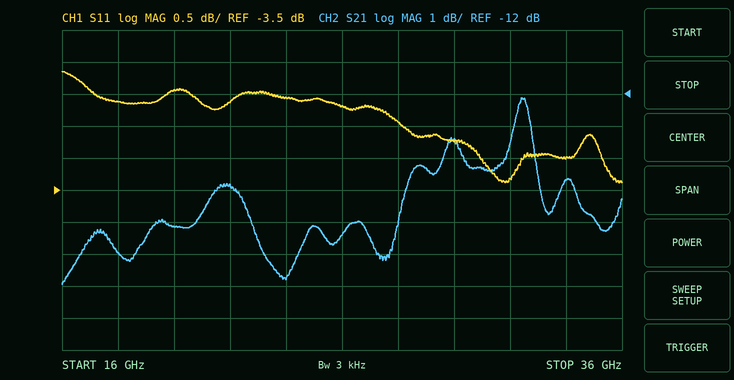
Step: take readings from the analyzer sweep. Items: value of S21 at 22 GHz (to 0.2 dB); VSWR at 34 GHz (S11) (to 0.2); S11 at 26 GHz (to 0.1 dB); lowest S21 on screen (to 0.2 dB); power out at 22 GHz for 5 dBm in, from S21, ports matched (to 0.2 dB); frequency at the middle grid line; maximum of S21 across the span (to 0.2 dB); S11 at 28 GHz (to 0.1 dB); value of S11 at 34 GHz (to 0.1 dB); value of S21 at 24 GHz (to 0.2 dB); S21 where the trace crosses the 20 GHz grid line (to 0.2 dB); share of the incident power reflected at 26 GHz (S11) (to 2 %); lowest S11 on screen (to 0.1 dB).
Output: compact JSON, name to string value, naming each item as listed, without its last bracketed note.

{"value of S21 at 22 GHz": "-14.8 dB", "VSWR at 34 GHz (S11)": "5.8", "S11 at 26 GHz": "-2.2 dB", "lowest S21 on screen": "-18.0 dB", "power out at 22 GHz for 5 dBm in, from S21, ports matched": "-9.8 dBm", "frequency at the middle grid line": "26 GHz", "maximum of S21 across the span": "-12.2 dB", "S11 at 28 GHz": "-2.4 dB", "value of S11 at 34 GHz": "-3.0 dB", "value of S21 at 24 GHz": "-17.8 dB", "S21 where the trace crosses the 20 GHz grid line": "-16.2 dB", "share of the incident power reflected at 26 GHz (S11)": "60 %", "lowest S11 on screen": "-3.4 dB"}
